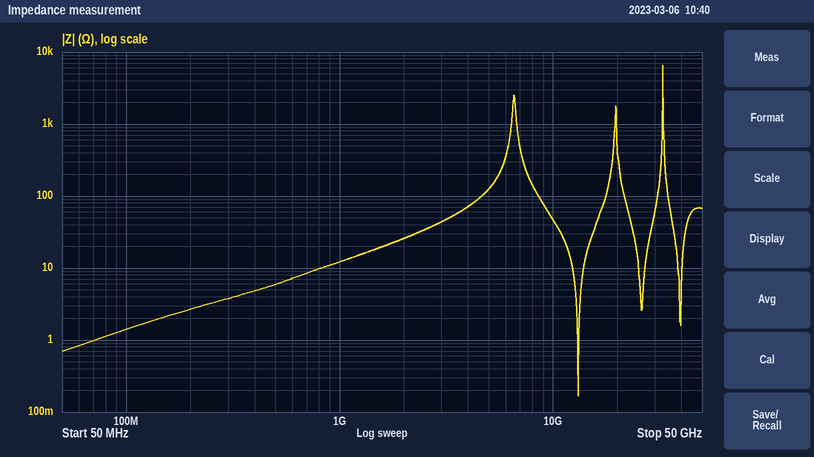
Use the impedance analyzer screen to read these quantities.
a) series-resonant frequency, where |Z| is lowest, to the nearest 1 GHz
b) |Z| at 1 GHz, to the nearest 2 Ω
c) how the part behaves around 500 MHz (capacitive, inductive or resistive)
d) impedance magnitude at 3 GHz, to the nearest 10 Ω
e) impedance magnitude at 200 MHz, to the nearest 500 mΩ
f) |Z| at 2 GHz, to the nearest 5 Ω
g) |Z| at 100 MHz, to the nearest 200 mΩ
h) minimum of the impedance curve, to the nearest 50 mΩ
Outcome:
13 GHz
12 Ω
inductive
40 Ω
2.5 Ω
25 Ω
1.4 Ω
150 mΩ
